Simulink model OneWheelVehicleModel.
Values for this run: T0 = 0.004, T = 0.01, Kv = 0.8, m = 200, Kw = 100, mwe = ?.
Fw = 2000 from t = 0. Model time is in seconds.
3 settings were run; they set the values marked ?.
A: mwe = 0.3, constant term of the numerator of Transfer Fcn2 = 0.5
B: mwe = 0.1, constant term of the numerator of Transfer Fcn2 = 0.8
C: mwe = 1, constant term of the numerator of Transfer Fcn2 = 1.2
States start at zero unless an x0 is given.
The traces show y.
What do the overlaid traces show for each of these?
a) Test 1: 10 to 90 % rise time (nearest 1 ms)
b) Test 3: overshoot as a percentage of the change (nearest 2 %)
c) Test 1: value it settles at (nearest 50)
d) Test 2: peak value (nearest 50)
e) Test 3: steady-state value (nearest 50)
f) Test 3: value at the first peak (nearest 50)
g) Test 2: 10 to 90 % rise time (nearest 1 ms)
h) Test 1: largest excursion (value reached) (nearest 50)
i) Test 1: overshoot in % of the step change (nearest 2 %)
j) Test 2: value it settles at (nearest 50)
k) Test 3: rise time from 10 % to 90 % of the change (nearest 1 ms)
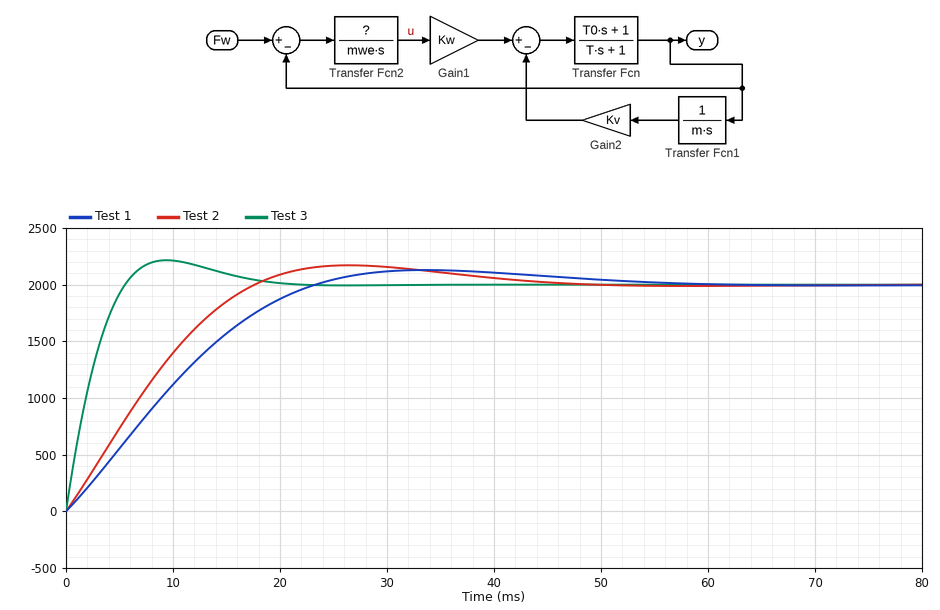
17 ms
10 %
2000
2150
2000
2200
13 ms
2150
6 %
2000
4 ms
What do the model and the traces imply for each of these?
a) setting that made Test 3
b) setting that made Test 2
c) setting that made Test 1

B
A
C
